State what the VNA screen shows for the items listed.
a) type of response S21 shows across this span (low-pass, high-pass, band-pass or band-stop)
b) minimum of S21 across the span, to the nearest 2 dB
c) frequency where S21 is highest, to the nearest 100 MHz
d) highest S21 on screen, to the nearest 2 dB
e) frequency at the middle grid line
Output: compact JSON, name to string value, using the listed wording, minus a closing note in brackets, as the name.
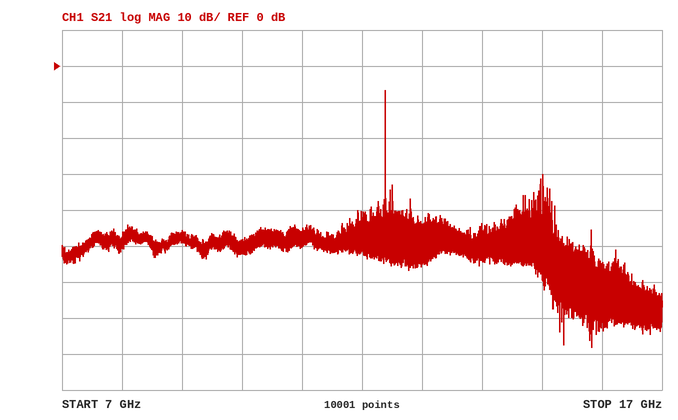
{"type of response S21 shows across this span": "band-pass", "minimum of S21 across the span, to the nearest 2 dB": "-78 dB", "frequency where S21 is highest, to the nearest 100 MHz": "12.4 GHz", "highest S21 on screen, to the nearest 2 dB": "-6 dB", "frequency at the middle grid line": "12 GHz"}
